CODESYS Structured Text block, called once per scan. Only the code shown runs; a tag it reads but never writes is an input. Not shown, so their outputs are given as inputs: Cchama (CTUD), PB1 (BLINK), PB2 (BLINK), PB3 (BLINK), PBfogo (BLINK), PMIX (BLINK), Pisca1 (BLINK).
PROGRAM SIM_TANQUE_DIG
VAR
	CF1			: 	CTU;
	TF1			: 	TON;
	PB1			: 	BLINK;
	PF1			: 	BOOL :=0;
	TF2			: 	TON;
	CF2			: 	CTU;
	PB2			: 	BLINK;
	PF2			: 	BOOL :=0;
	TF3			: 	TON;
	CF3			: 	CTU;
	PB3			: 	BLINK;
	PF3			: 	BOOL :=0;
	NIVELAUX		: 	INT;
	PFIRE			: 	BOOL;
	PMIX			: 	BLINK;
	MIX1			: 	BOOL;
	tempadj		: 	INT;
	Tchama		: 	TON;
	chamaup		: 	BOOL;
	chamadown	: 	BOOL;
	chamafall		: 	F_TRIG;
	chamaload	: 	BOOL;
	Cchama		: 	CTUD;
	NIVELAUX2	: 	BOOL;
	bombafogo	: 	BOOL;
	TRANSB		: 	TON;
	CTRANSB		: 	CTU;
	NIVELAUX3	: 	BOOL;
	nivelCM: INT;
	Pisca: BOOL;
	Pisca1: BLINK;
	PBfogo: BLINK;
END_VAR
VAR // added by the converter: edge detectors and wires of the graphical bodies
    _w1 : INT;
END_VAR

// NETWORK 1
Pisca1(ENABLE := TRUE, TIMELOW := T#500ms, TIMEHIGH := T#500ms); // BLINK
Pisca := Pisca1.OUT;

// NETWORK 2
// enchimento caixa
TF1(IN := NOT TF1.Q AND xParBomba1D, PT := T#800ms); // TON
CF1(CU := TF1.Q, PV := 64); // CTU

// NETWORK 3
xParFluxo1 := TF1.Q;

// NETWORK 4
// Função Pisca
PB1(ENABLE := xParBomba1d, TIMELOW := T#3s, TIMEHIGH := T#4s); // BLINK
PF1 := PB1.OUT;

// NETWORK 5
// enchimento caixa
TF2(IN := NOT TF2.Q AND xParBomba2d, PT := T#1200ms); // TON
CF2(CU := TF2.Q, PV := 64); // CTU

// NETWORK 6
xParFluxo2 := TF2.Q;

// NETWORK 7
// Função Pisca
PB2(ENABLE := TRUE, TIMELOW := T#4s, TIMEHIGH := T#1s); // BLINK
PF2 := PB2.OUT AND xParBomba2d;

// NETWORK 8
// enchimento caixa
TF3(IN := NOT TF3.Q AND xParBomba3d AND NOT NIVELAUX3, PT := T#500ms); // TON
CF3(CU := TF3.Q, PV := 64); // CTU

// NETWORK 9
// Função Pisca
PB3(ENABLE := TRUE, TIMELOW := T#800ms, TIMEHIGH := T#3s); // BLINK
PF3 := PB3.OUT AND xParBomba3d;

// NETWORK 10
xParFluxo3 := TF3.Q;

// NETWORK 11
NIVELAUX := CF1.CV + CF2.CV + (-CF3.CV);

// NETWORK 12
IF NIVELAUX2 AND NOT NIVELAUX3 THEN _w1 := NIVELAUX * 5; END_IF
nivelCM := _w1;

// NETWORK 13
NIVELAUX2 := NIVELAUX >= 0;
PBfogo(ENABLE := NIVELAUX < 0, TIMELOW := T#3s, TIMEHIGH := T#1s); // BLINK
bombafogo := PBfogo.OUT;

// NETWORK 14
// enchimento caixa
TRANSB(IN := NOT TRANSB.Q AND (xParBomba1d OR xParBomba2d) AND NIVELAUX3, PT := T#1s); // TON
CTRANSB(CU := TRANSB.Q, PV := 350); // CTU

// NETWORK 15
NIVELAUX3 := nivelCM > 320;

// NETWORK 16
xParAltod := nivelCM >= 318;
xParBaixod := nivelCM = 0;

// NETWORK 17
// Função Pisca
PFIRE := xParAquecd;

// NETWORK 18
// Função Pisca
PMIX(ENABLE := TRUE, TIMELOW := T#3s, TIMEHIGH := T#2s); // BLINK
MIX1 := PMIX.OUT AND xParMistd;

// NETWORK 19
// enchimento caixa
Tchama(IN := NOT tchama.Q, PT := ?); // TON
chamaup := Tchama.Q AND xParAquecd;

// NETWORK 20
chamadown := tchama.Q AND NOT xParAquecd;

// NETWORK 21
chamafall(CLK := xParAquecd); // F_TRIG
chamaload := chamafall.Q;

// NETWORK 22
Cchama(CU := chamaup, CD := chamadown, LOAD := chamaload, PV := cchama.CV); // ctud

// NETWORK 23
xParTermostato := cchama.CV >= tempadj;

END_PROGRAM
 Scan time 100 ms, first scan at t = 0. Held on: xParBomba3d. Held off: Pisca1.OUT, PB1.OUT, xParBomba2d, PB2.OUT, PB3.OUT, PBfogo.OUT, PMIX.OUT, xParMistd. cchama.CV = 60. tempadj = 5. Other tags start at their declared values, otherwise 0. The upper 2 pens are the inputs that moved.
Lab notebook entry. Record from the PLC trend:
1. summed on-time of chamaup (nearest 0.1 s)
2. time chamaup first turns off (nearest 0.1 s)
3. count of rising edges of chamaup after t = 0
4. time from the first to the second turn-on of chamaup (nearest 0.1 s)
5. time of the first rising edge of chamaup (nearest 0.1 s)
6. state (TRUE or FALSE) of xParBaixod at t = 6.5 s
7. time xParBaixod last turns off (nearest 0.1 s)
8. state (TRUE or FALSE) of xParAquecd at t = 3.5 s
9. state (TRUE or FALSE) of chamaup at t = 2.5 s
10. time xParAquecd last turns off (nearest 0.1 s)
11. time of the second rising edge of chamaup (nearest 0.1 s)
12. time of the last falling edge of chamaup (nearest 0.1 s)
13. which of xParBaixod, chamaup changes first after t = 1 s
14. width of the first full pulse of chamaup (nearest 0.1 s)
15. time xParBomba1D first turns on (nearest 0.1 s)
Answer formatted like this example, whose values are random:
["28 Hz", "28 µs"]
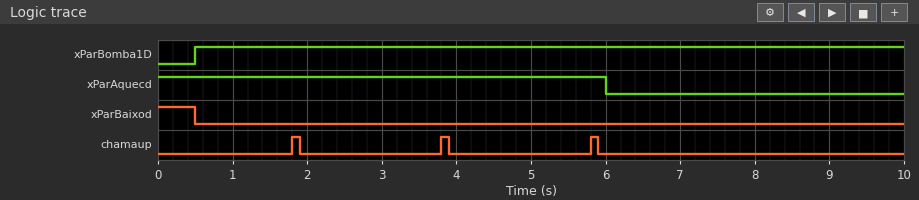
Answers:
["0.3 s", "1.9 s", "3", "2.0 s", "1.8 s", "FALSE", "0.5 s", "TRUE", "FALSE", "6.0 s", "3.8 s", "5.9 s", "chamaup", "0.1 s", "0.5 s"]
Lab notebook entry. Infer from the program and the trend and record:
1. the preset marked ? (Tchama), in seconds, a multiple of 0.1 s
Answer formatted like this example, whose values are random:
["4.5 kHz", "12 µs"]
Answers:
["1.8 s"]
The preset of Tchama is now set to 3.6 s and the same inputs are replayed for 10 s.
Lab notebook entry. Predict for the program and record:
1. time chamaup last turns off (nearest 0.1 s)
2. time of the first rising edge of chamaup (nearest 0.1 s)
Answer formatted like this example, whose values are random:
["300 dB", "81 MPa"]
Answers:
["3.7 s", "3.6 s"]
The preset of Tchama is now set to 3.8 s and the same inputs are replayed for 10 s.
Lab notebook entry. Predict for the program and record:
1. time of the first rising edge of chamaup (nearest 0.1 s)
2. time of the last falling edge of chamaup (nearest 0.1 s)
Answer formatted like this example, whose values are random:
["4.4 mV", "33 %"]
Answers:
["3.8 s", "3.9 s"]
